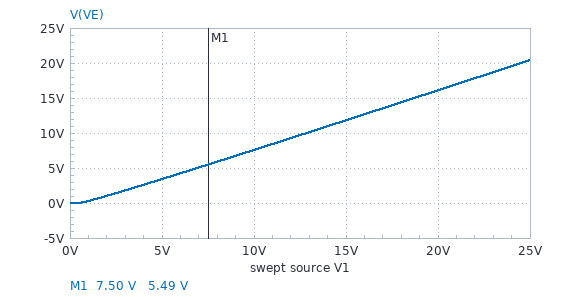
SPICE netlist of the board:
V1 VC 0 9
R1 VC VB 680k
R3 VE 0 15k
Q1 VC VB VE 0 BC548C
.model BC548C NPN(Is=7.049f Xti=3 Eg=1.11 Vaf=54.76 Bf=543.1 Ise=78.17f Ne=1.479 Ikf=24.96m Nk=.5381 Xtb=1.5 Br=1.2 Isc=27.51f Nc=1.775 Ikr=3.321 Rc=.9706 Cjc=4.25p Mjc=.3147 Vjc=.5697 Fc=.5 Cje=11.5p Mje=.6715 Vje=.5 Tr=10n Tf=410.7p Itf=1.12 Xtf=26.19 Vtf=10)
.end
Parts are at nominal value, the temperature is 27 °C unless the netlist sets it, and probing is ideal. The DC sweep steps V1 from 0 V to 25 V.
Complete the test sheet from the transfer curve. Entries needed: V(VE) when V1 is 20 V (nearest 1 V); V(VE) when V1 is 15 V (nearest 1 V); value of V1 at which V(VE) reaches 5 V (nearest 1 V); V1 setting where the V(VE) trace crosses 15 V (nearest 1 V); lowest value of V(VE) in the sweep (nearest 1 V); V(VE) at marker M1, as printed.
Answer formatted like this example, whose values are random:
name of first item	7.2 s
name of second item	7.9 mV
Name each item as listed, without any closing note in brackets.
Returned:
V(VE) when V1 is 20 V	16 V
V(VE) when V1 is 15 V	12 V
value of V1 at which V(VE) reaches 5 V	7 V
V1 setting where the V(VE) trace crosses 15 V	19 V
lowest value of V(VE) in the sweep	0 V
V(VE) at marker M1, as printed	5.49 V
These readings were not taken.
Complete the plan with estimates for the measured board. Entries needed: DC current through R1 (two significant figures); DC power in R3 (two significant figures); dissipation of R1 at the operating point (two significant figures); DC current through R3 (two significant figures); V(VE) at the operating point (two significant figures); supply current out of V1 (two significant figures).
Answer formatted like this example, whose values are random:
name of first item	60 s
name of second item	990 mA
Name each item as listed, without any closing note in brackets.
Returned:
DC current through R1	2.4 µA
DC power in R3	3.0 mW
dissipation of R1 at the operating point	3.8 µW
DC current through R3	450 µA
V(VE) at the operating point	6.7 V
supply current out of V1	450 µA
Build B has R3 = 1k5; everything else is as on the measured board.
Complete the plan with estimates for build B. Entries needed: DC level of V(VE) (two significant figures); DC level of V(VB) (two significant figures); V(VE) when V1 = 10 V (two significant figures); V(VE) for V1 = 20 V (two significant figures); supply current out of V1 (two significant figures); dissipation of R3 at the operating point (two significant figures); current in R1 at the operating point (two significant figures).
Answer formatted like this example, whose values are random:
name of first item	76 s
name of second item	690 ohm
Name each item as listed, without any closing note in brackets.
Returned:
DC level of V(VE)	3.0 V
DC level of V(VB)	3.7 V
V(VE) when V1 = 10 V	3.4 V
V(VE) for V1 = 20 V	7.6 V
supply current out of V1	2.0 mA
dissipation of R3 at the operating point	5.9 mW
current in R1 at the operating point	7.8 µA
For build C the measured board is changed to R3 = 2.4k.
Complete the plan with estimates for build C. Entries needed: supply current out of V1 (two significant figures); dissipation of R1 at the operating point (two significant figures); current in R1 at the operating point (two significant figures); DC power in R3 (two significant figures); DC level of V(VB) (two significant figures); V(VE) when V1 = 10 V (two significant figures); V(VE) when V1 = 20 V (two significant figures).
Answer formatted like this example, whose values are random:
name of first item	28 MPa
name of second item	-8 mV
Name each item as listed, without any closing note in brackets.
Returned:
supply current out of V1	1.6 mA
dissipation of R1 at the operating point	29 µW
current in R1 at the operating point	6.6 µA
DC power in R3	6.2 mW
DC level of V(VB)	4.5 V
V(VE) when V1 = 10 V	4.4 V
V(VE) when V1 = 20 V	9.7 V
